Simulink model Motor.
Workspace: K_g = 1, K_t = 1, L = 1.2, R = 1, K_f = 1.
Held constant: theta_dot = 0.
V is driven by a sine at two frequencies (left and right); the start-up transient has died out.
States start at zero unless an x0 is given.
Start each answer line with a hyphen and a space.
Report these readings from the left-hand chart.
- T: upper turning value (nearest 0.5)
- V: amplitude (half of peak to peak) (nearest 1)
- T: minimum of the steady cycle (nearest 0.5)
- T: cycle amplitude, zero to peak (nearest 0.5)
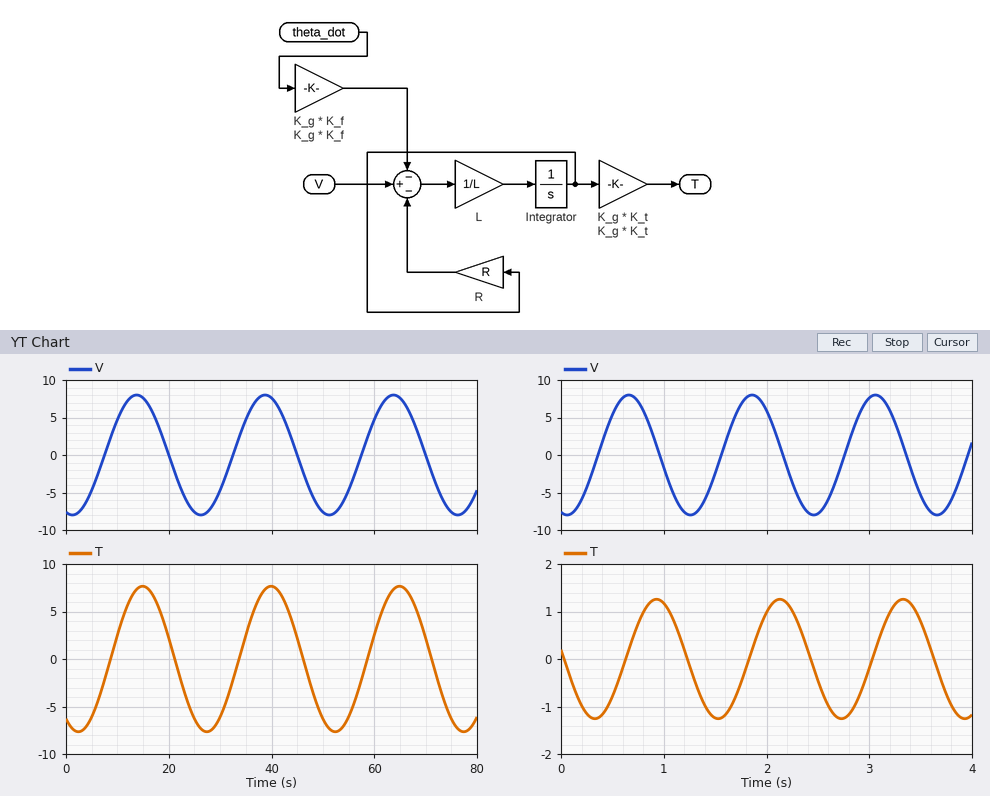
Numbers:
- 7.5
- 8
- -7.5
- 7.5
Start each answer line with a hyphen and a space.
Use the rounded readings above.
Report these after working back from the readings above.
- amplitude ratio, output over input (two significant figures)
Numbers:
- 0.94
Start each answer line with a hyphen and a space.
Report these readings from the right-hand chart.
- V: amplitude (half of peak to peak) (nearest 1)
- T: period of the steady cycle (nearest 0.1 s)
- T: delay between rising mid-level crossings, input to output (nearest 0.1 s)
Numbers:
- 8
- 1.2 s
- 0.3 s
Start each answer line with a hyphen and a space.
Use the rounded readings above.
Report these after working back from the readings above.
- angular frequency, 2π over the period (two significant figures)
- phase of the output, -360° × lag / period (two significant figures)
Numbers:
- 5.2 rad/s
- -90°
